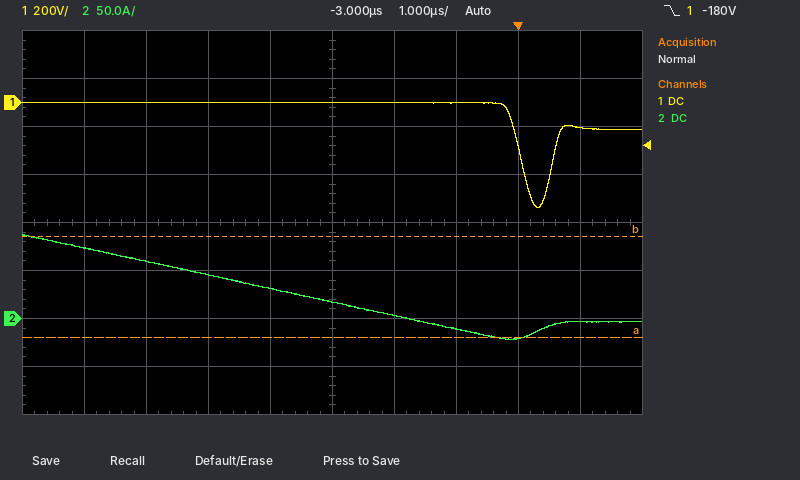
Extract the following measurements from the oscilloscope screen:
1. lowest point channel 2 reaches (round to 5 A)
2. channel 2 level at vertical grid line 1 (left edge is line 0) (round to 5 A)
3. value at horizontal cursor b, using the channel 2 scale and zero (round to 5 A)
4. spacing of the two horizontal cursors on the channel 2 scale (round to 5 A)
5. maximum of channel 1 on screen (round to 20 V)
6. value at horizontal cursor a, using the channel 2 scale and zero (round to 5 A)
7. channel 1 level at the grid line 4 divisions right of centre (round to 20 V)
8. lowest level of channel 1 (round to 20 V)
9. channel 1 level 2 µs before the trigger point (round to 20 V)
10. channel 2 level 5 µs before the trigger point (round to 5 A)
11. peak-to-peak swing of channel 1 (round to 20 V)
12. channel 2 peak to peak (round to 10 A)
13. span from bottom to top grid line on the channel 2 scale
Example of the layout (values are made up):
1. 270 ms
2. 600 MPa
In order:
1. -20 A
2. 75 A
3. 85 A
4. 105 A
5. 0 V
6. -20 A
7. -100 V
8. -440 V
9. 0 V
10. 45 A
11. 440 V
12. 110 A
13. 400 A
